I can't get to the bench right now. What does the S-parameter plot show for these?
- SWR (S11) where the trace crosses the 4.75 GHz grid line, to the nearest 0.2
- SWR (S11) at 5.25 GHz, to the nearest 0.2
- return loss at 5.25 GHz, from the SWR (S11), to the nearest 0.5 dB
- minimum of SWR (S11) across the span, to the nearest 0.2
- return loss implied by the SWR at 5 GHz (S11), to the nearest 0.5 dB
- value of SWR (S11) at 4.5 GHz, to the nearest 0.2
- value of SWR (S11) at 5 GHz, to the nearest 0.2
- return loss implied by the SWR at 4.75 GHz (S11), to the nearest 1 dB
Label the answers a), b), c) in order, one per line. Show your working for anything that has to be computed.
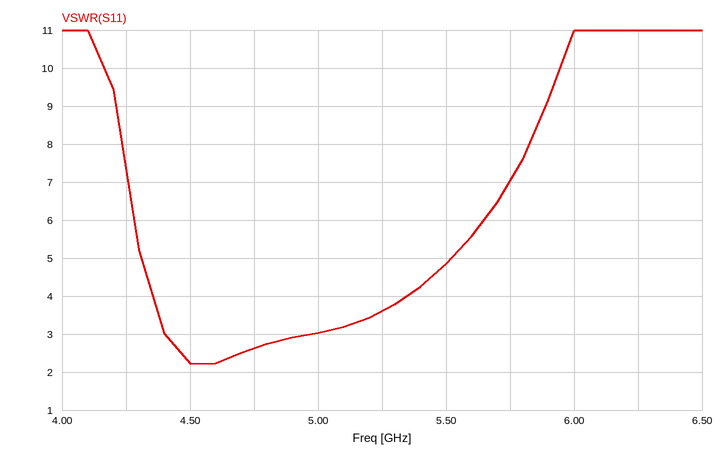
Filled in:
a) 2.6
b) 3.6
c) −20 log10((3.6 − 1)/(3.6 + 1)) ≈ 5.0 dB
d) 2.2
e) −20 log10((3 − 1)/(3 + 1)) ≈ 6.0 dB
f) 2.2
g) 3.0
h) −20 log10((2.6 − 1)/(2.6 + 1)) ≈ 7 dB
